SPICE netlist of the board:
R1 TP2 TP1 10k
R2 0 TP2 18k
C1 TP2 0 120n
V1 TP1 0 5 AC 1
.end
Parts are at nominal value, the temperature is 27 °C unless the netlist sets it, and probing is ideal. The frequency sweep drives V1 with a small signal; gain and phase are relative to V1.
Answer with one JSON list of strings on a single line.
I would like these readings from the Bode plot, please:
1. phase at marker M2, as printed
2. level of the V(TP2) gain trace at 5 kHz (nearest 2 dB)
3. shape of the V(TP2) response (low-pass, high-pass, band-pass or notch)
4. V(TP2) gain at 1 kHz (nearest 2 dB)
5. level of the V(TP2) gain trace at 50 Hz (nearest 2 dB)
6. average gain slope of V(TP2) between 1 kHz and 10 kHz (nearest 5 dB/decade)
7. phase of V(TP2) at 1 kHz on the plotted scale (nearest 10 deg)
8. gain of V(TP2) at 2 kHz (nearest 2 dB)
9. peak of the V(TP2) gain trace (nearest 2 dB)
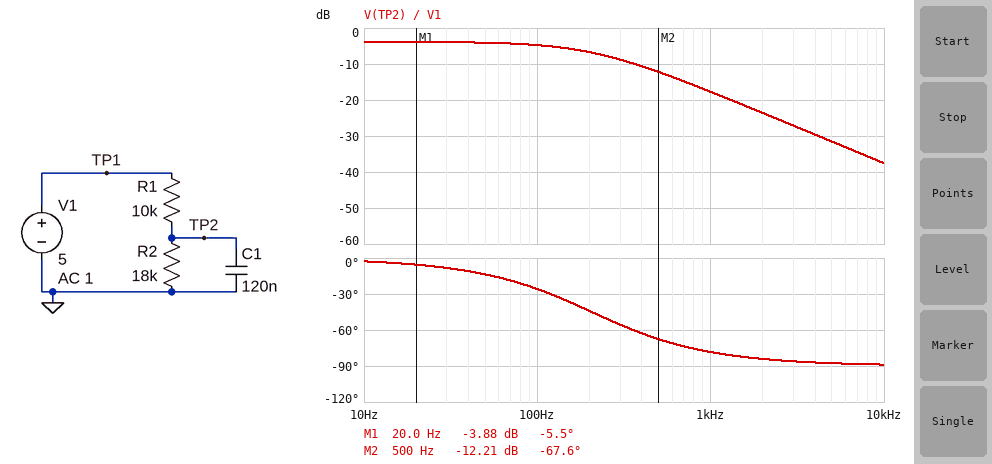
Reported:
["-67.6 deg", "-32 dB", "low-pass", "-18 dB", "-4 dB", "-20 dB/decade", "-80 deg", "-24 dB", "-4 dB"]
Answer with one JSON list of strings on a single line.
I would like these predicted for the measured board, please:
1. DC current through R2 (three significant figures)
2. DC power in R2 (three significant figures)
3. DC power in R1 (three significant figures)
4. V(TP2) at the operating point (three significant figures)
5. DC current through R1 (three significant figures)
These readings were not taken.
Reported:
["179 µA", "574 µW", "319 µW", "3.21 V", "179 µA"]
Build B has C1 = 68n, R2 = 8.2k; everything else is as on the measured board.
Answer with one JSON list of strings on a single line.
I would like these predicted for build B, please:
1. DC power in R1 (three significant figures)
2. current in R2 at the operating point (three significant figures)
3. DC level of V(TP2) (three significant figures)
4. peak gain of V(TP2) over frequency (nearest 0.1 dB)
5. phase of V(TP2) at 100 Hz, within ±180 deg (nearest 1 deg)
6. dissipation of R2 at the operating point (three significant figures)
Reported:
["755 µW", "275 µA", "2.25 V", "-6.9 dB", "-11 deg", "619 µW"]
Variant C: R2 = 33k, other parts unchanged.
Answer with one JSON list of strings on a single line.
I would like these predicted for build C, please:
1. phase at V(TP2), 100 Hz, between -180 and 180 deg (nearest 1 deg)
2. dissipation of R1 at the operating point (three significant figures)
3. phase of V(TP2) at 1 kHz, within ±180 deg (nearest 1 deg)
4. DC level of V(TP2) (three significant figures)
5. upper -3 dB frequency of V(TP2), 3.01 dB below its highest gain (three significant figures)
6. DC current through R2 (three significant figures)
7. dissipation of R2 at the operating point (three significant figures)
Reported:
["-30 deg", "135 µW", "-80 deg", "3.84 V", "173 Hz", "116 µA", "446 µW"]
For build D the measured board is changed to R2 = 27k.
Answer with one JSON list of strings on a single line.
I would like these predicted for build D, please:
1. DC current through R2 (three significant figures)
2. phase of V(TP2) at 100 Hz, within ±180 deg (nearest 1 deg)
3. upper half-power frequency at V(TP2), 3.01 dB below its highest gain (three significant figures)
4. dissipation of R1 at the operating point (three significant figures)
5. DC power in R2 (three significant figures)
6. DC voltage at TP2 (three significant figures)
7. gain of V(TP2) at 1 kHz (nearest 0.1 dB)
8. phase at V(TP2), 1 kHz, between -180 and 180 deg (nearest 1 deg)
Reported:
["135 µA", "-29 deg", "182 Hz", "183 µW", "493 µW", "3.65 V", "-17.7 dB", "-80 deg"]
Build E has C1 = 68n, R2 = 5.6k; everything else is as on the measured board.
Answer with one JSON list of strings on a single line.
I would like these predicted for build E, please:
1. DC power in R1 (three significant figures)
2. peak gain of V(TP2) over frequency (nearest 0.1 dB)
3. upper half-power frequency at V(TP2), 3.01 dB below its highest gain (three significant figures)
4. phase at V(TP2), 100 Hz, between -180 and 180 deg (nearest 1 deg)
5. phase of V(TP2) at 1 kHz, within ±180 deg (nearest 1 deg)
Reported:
["1.03 mW", "-8.9 dB", "652 Hz", "-9 deg", "-57 deg"]
